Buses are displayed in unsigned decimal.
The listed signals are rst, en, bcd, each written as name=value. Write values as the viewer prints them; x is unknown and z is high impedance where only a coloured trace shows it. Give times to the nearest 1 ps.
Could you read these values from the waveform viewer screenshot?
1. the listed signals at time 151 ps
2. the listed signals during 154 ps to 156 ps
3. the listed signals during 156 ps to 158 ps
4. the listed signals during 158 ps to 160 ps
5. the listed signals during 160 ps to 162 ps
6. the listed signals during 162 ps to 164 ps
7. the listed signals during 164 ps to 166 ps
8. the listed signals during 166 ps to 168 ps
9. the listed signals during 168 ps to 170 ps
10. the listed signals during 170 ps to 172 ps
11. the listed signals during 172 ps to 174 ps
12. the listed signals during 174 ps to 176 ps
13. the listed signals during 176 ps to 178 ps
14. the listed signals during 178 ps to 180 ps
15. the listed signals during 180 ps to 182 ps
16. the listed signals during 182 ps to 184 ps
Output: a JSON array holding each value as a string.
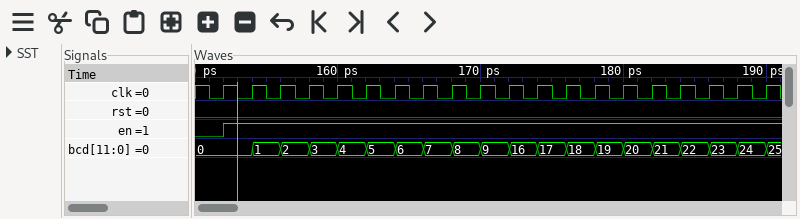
["rst=0, en=0, bcd=0", "rst=0, en=1, bcd=1", "rst=0, en=1, bcd=2", "rst=0, en=1, bcd=3", "rst=0, en=1, bcd=4", "rst=0, en=1, bcd=5", "rst=0, en=1, bcd=6", "rst=0, en=1, bcd=7", "rst=0, en=1, bcd=8", "rst=0, en=1, bcd=9", "rst=0, en=1, bcd=16", "rst=0, en=1, bcd=17", "rst=0, en=1, bcd=18", "rst=0, en=1, bcd=19", "rst=0, en=1, bcd=20", "rst=0, en=1, bcd=21"]
